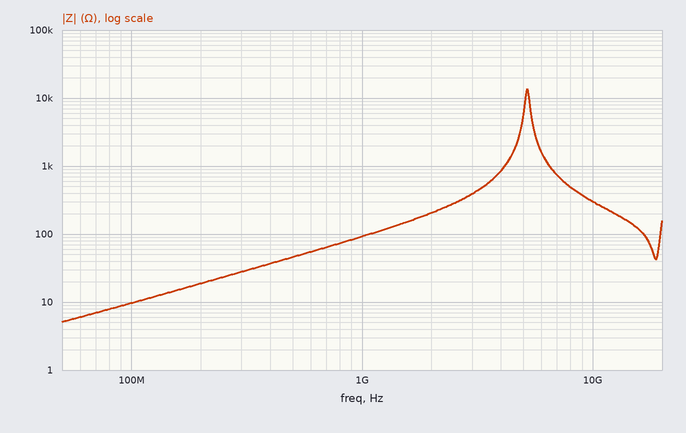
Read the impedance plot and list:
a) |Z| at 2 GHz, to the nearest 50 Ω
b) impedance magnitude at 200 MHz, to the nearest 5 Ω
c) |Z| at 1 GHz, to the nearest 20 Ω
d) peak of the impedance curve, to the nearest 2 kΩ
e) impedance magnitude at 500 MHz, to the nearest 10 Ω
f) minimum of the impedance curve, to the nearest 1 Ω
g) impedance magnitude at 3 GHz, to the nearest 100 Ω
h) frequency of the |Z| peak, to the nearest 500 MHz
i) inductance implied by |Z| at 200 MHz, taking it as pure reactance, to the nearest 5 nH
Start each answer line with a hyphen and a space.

- 200 Ω
- 20 Ω
- 100 Ω
- 14 kΩ
- 50 Ω
- 5 Ω
- 400 Ω
- 5.0 GHz
- 15 nH
